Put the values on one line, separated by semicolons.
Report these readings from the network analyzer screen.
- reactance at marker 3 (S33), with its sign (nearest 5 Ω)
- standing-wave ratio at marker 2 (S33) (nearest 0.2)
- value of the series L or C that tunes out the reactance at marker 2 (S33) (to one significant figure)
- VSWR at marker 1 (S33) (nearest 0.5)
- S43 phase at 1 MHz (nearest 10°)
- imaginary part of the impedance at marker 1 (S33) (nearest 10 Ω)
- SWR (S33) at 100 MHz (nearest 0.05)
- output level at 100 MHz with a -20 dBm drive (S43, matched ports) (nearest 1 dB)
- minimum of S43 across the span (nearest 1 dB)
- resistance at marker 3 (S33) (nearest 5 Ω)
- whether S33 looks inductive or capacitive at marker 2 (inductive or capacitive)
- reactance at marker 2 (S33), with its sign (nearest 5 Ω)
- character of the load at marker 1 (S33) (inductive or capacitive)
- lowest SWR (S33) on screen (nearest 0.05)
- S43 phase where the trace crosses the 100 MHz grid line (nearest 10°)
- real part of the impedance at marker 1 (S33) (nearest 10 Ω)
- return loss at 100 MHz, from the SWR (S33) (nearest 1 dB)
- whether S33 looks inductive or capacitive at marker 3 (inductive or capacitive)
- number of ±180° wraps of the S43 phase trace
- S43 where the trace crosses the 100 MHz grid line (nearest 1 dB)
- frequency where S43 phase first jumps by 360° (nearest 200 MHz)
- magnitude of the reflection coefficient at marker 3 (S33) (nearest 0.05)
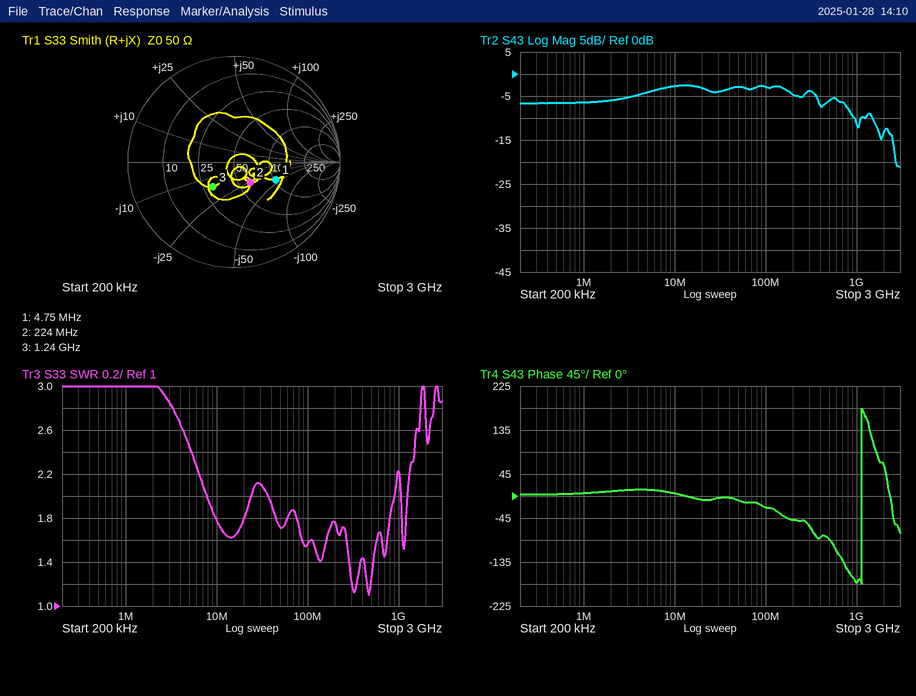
-15 Ω; 1.6; 20 nH; 2.5; 10°; -40 Ω; 1.55; -23 dBm; -21 dB; 30 Ω; capacitive; -25 Ω; capacitive; 1.10; -20°; 100 Ω; 13 dB; capacitive; 1; -3 dB; 1.2 GHz; 0.30
